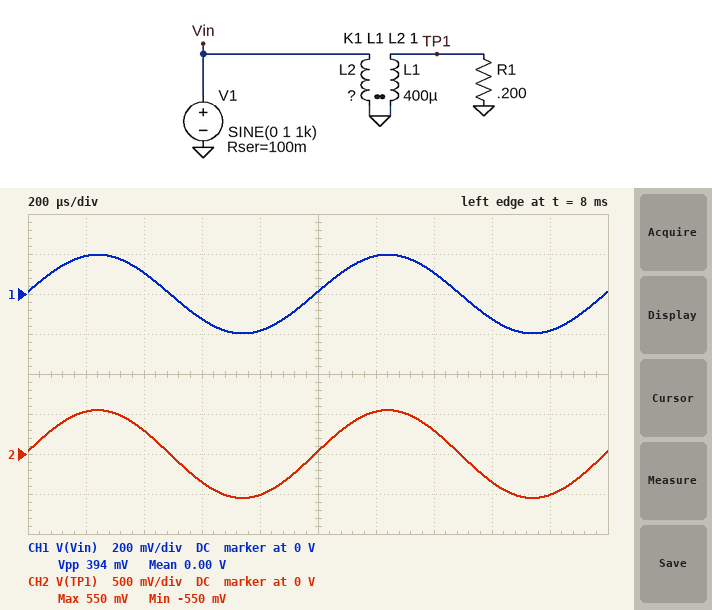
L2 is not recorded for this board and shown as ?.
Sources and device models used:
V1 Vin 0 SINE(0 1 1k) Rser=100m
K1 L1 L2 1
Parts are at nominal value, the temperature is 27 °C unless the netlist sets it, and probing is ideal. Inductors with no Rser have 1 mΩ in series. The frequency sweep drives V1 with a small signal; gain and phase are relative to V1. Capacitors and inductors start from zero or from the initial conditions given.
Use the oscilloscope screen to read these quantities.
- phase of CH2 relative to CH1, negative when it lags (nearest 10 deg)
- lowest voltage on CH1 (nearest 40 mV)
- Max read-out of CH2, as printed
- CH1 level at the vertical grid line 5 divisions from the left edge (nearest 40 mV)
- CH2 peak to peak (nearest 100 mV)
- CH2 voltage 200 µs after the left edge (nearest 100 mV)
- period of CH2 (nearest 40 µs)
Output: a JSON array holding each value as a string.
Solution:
["0 deg", "-200 mV", "550 mV", "0 V", "1.1 V", "500 mV", "1.00 ms"]
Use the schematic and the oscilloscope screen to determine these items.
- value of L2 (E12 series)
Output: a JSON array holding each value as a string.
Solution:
["47 µH"]
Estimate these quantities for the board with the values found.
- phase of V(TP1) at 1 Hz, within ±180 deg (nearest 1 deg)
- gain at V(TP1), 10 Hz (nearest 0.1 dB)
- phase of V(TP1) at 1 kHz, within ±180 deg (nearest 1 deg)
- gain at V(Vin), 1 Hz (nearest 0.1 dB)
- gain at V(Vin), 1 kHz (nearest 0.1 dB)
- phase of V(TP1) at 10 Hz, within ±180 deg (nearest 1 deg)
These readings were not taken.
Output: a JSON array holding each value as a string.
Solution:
["89 deg", "-21.5 dB", "4 deg", "-39.7 dB", "-14.1 dB", "81 deg"]
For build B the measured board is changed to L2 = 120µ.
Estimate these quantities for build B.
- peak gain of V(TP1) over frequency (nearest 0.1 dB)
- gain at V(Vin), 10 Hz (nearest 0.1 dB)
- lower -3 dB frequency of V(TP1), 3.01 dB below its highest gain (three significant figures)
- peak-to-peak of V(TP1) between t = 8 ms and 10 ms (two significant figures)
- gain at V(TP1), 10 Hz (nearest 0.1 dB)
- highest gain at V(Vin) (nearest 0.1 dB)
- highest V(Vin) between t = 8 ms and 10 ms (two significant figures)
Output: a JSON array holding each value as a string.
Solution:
["-3.4 dB", "-22.5 dB", "50.1 Hz", "1.4 V", "-17.5 dB", "-8.4 dB", "380 mV"]
